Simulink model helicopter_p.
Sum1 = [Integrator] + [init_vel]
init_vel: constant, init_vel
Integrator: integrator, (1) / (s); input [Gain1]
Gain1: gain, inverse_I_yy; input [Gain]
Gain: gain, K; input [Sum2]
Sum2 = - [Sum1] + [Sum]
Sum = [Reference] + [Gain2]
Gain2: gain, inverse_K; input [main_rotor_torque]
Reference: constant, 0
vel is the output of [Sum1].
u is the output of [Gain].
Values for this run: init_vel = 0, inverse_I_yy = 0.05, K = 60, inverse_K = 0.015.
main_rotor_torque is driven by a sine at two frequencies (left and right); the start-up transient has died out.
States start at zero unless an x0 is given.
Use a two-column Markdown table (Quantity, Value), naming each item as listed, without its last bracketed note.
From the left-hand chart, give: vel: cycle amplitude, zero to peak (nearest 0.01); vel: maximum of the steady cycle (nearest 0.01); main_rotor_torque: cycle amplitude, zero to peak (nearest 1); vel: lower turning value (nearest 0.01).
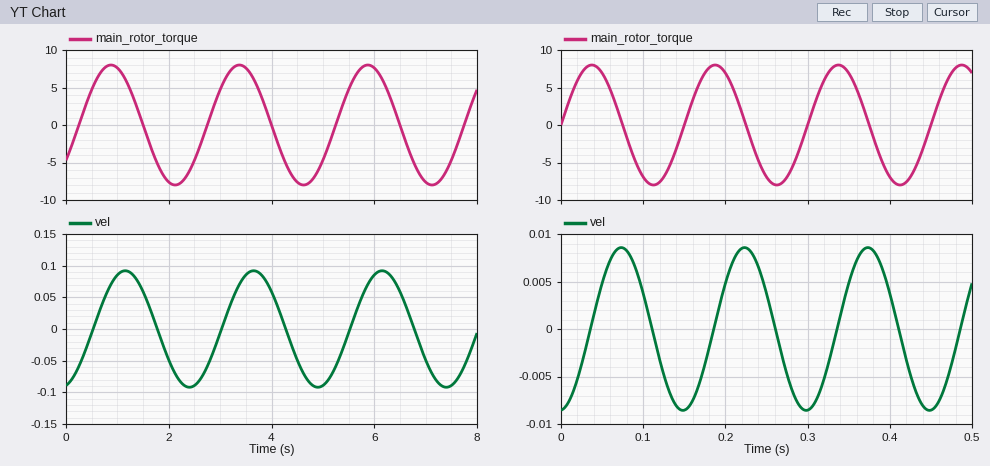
| Quantity | Value |
|---|---|
| vel: cycle amplitude, zero to peak | 0.09 |
| vel: maximum of the steady cycle | 0.09 |
| main_rotor_torque: cycle amplitude, zero to peak | 8 |
| vel: lower turning value | -0.09 |
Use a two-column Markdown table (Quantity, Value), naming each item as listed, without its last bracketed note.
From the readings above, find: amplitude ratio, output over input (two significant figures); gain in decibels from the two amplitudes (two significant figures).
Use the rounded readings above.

| Quantity | Value |
|---|---|
| amplitude ratio, output over input | 0.011 |
| gain in decibels from the two amplitudes | -39 dB |
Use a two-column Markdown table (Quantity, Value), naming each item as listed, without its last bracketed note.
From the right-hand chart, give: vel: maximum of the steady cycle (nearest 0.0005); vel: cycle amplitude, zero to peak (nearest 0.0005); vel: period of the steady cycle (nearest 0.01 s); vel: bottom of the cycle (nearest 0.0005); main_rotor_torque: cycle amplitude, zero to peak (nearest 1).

| Quantity | Value |
|---|---|
| vel: maximum of the steady cycle | 0.0085 |
| vel: cycle amplitude, zero to peak | 0.0085 |
| vel: period of the steady cycle | 0.15 s |
| vel: bottom of the cycle | -0.0085 |
| main_rotor_torque: cycle amplitude, zero to peak | 8 |
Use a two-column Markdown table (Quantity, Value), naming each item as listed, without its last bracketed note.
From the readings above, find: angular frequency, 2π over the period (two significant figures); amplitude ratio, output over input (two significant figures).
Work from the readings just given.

| Quantity | Value |
|---|---|
| angular frequency, 2π over the period | 42 rad/s |
| amplitude ratio, output over input | 0.0011 |
